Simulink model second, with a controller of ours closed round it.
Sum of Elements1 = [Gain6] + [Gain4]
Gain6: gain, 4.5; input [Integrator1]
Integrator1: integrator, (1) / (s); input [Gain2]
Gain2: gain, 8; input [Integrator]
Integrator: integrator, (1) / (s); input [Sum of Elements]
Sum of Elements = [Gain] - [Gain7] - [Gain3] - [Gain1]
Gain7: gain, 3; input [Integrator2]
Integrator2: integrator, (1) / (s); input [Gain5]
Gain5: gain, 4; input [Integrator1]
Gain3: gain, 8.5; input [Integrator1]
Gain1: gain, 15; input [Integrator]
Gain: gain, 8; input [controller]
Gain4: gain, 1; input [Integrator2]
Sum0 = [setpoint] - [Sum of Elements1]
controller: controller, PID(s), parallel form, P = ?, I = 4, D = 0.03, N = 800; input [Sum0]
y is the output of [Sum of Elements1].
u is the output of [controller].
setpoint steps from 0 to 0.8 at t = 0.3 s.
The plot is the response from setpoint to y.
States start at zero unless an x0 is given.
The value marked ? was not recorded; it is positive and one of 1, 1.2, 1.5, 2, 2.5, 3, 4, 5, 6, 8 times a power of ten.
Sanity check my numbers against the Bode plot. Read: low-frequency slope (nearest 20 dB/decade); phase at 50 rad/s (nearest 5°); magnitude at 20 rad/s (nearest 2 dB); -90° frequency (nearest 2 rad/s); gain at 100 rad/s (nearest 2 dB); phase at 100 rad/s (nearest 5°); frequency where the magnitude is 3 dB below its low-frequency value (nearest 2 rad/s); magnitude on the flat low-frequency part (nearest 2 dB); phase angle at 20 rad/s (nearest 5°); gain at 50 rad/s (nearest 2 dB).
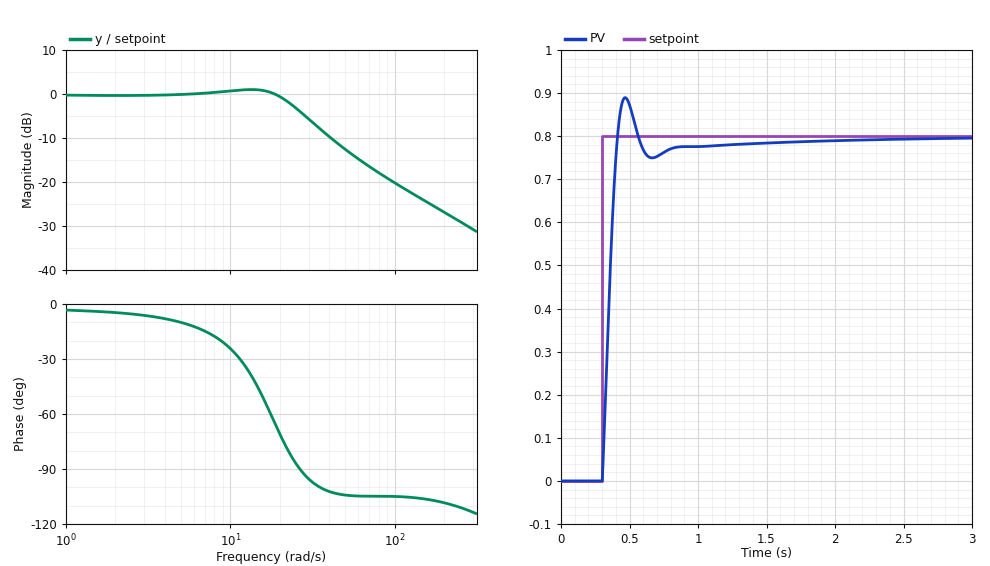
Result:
0 dB/decade
-105°
0 dB
26 rad/s
-20 dB
-105°
26 rad/s
0 dB
-70°
-12 dB
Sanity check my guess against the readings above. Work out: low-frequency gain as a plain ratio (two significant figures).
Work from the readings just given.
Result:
1.0
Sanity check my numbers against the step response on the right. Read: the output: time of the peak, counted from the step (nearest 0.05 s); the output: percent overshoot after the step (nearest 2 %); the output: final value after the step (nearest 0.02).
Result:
0.15 s
12 %
0.80
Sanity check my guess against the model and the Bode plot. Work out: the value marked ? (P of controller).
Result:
1.2
